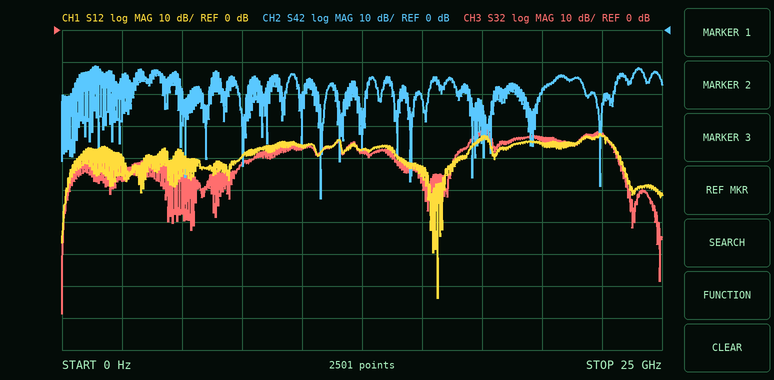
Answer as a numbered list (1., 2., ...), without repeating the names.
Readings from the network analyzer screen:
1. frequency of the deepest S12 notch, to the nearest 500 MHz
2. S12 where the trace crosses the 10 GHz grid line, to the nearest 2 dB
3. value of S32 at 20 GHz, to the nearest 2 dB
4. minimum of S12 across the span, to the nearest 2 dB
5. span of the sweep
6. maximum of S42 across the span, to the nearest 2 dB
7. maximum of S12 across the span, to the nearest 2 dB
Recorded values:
1. 15.5 GHz
2. -36 dB
3. -34 dB
4. -84 dB
5. 25 GHz
6. -12 dB
7. -32 dB
